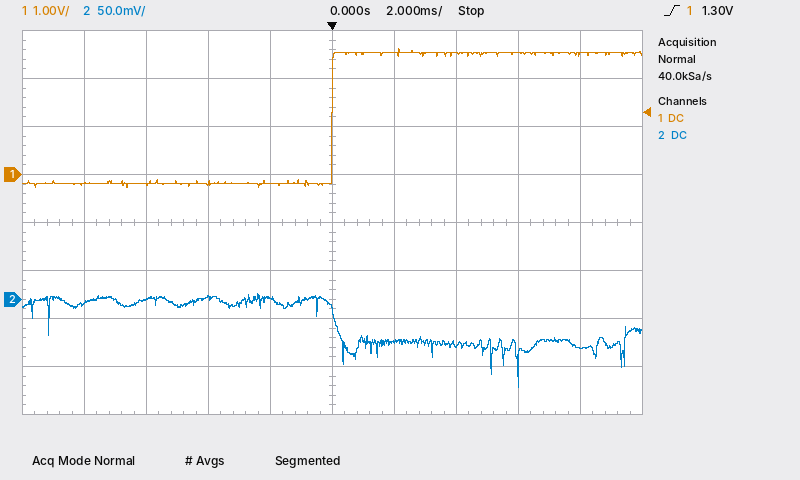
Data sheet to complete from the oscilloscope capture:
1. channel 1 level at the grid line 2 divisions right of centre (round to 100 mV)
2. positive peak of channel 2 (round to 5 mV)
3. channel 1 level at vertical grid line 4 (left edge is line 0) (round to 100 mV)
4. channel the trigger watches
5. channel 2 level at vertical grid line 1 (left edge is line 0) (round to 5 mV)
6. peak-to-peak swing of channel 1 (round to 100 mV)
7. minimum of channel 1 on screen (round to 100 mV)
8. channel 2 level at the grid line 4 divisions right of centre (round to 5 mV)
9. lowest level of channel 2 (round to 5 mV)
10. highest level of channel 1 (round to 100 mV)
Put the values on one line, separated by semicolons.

2.5 V; 5 mV; -200 mV; channel 1; -5 mV; 2.9 V; -300 mV; -50 mV; -90 mV; 2.6 V
